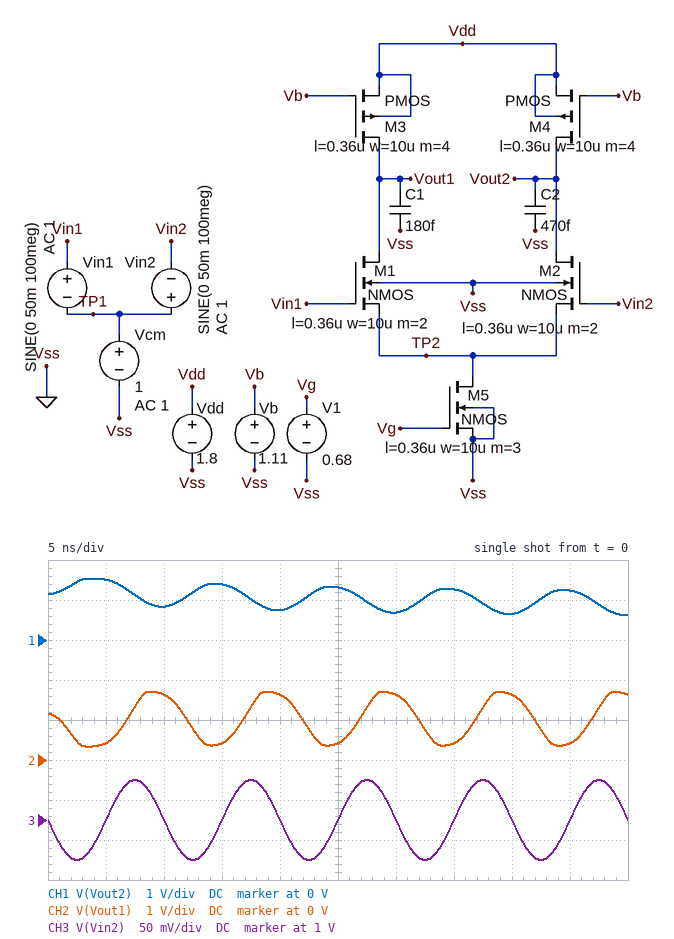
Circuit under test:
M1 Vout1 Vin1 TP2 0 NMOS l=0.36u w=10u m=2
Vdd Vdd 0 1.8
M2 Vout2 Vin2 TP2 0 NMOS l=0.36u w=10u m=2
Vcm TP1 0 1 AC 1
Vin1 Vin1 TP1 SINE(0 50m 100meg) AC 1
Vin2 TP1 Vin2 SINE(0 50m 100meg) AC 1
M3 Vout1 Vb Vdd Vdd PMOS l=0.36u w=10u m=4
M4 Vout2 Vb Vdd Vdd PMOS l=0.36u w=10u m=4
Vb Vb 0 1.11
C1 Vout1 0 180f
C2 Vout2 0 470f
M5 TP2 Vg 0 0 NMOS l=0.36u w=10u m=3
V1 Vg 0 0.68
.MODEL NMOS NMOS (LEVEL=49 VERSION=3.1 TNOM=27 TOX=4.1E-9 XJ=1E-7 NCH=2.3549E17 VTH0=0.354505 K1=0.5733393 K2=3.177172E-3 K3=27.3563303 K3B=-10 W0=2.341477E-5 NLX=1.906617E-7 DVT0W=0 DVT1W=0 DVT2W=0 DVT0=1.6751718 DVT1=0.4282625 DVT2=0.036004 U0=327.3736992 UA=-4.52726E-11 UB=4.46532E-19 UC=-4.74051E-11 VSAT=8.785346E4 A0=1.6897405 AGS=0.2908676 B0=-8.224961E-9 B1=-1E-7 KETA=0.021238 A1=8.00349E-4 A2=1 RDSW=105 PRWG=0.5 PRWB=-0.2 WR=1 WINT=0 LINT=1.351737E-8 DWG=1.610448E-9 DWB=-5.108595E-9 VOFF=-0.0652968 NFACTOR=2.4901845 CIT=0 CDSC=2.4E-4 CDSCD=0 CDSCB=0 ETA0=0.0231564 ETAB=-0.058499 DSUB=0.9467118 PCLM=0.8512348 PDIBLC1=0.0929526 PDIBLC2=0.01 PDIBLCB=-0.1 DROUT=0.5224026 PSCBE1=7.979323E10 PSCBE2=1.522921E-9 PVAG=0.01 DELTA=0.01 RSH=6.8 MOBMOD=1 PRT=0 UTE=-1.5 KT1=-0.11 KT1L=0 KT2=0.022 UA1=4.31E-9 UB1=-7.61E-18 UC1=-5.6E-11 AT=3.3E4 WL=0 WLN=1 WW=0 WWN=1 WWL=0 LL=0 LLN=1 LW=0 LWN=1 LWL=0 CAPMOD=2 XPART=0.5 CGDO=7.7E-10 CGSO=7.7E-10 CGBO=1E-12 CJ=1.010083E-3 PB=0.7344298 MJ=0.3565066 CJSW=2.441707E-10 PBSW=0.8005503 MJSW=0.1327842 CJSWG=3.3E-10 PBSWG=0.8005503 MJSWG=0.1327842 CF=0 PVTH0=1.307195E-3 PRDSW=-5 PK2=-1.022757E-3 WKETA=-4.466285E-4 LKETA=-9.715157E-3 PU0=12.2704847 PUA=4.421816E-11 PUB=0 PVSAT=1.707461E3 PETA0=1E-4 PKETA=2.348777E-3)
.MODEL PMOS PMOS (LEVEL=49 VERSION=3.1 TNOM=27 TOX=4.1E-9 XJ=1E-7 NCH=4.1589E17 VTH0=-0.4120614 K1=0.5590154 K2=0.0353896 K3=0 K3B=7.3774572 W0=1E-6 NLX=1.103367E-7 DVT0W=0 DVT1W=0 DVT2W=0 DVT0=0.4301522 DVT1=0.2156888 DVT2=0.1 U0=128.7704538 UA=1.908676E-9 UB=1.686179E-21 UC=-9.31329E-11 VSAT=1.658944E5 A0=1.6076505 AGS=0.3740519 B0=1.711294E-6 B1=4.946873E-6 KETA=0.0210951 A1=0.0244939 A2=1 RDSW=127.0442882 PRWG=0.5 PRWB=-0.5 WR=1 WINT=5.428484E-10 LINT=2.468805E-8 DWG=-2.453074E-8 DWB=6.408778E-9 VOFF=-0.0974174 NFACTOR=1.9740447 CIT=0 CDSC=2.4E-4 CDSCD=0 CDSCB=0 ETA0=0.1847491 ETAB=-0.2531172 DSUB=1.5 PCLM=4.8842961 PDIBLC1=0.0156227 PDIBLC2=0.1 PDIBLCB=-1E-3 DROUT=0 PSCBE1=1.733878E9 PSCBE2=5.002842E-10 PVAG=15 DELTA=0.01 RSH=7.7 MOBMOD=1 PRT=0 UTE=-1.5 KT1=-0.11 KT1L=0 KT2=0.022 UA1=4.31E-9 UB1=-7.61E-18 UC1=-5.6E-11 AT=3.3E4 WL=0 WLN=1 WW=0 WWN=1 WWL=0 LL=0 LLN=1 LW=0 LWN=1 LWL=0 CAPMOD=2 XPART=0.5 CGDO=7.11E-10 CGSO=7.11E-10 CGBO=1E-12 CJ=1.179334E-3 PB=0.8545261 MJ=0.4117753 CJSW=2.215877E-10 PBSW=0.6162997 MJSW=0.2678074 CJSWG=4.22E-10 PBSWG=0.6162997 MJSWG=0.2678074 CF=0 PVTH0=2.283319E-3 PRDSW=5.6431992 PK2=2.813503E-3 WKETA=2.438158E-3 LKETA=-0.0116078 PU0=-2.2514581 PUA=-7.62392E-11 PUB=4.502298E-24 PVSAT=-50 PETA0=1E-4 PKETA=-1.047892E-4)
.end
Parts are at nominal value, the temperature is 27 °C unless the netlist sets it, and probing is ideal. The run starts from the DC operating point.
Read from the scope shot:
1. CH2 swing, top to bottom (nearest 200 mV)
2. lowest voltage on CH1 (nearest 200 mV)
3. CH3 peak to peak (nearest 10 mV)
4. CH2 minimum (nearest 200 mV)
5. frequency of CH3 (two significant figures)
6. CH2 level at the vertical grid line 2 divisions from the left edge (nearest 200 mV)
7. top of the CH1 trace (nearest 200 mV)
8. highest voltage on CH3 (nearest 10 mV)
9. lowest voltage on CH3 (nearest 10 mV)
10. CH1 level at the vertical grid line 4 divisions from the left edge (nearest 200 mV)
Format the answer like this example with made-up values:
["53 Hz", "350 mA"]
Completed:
["1.4 V", "600 mV", "100 mV", "400 mV", "100 MHz", "1.6 V", "1.6 V", "1.05 V", "950 mV", "800 mV"]
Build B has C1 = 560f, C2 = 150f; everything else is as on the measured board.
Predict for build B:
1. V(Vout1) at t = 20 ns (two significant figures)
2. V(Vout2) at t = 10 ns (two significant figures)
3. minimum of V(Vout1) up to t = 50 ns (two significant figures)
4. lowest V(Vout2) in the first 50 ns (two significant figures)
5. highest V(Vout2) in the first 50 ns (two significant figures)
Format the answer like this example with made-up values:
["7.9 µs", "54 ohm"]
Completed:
["1.1 V", "420 mV", "580 mV", "340 mV", "1.7 V"]
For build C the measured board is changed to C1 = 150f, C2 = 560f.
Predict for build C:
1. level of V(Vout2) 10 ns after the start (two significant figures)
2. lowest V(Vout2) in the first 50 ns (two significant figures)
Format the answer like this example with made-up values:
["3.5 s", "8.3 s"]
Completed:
["870 mV", "590 mV"]
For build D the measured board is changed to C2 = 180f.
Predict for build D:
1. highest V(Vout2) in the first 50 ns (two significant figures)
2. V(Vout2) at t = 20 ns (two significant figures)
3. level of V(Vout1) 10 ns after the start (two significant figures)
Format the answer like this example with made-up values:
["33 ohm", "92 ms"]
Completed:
["1.7 V", "420 mV", "1.6 V"]
